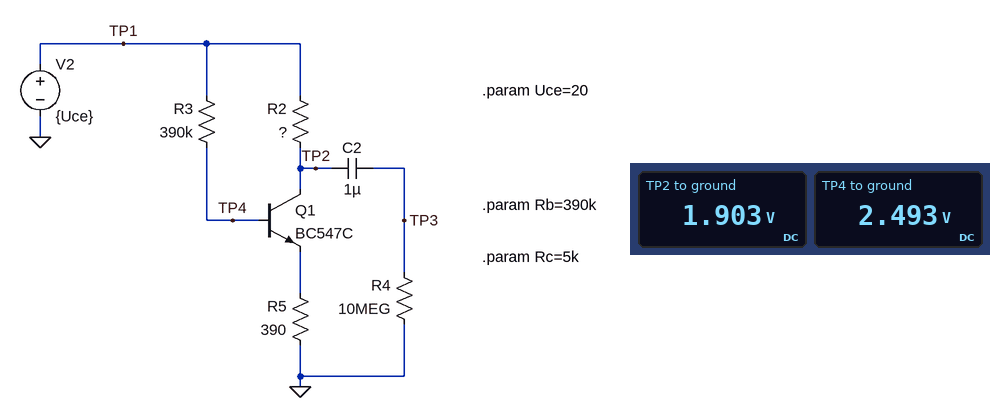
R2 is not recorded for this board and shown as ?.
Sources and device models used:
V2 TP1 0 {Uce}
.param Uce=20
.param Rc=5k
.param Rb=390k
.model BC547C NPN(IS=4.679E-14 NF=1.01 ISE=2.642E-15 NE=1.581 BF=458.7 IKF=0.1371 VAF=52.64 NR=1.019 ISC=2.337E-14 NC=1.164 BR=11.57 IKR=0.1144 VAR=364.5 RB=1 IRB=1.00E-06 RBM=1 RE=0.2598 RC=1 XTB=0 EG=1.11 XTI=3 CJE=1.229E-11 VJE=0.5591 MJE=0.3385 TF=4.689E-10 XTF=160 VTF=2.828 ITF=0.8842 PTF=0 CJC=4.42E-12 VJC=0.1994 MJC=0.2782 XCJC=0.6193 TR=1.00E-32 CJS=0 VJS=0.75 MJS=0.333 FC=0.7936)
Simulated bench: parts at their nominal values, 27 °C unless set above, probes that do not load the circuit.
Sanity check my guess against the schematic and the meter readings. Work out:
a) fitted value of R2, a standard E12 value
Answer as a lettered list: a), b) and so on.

a) 3.9 kΩ
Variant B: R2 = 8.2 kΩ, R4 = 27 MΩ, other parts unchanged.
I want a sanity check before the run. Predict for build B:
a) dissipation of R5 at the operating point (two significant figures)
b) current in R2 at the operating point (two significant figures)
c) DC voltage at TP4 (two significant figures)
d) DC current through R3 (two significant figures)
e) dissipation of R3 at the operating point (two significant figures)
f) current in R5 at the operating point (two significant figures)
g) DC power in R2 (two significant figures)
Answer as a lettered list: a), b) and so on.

a) 2.2 mW
b) 2.3 mA
c) 1.6 V
d) 47 µA
e) 870 µW
f) 2.4 mA
g) 44 mW
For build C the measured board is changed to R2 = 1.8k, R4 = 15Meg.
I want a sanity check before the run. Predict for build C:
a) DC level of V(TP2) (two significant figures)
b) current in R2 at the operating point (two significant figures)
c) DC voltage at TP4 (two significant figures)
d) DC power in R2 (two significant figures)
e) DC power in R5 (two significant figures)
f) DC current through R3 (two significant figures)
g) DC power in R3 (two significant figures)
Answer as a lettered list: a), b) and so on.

a) 3.7 V
b) 9.1 mA
c) 4.2 V
d) 150 mW
e) 32 mW
f) 40 µA
g) 640 µW
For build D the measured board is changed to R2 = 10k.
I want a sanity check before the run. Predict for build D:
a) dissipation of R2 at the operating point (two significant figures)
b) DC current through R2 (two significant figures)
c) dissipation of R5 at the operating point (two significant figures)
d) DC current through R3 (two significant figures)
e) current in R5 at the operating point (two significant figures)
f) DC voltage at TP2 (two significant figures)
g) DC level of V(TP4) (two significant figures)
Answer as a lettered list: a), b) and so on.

a) 37 mW
b) 1.9 mA
c) 1.5 mW
d) 48 µA
e) 2.0 mA
f) 810 mV
g) 1.4 V
